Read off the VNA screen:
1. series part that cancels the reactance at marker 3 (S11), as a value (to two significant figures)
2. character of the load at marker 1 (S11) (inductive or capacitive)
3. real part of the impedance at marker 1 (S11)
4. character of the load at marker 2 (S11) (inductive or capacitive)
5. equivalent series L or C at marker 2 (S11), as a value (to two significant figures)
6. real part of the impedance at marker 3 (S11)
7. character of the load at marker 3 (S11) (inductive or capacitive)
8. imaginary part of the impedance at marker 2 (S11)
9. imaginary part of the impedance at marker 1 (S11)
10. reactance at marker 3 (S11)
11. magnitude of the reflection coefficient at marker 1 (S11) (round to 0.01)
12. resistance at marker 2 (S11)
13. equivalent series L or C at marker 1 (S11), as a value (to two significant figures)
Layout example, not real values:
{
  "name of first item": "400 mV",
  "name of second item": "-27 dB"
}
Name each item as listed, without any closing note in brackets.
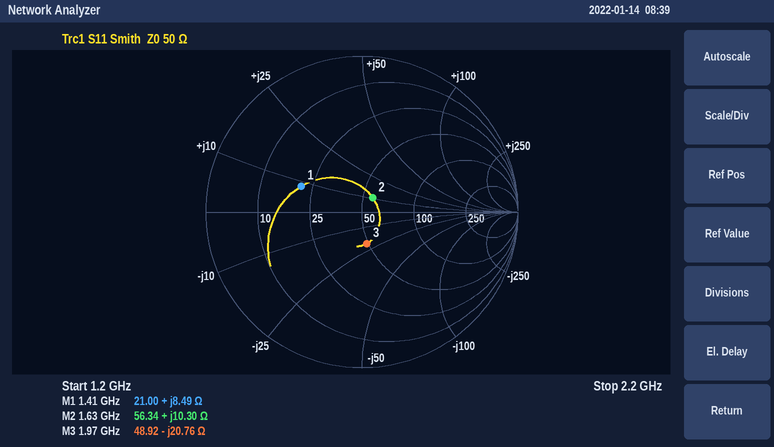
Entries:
{
  "series part that cancels the reactance at marker 3 (S11), as a value": "1.7 nH",
  "character of the load at marker 1 (S11)": "inductive",
  "real part of the impedance at marker 1": "21.00 Ω",
  "character of the load at marker 2 (S11)": "inductive",
  "equivalent series L or C at marker 2 (S11), as a value": "1.0 nH",
  "real part of the impedance at marker 3": "48.92 Ω",
  "character of the load at marker 3 (S11)": "capacitive",
  "imaginary part of the impedance at marker 2": "+10.30 Ω",
  "imaginary part of the impedance at marker 1": "+8.49 Ω",
  "reactance at marker 3": "-20.76 Ω",
  "magnitude of the reflection coefficient at marker 1 (S11)": "0.42",
  "resistance at marker 2": "56.34 Ω",
  "equivalent series L or C at marker 1 (S11), as a value": "960 pH"
}
